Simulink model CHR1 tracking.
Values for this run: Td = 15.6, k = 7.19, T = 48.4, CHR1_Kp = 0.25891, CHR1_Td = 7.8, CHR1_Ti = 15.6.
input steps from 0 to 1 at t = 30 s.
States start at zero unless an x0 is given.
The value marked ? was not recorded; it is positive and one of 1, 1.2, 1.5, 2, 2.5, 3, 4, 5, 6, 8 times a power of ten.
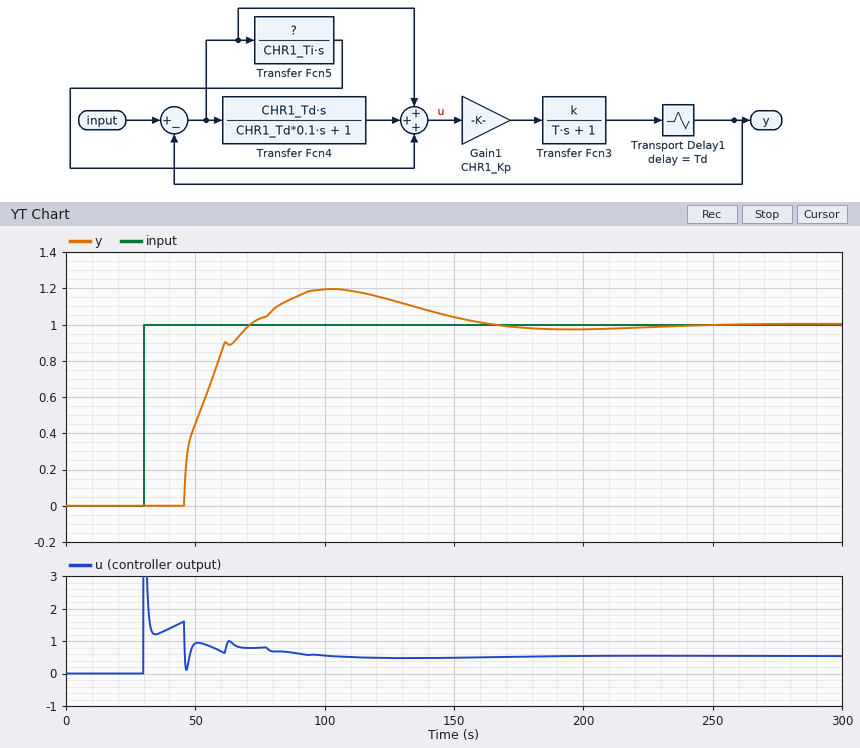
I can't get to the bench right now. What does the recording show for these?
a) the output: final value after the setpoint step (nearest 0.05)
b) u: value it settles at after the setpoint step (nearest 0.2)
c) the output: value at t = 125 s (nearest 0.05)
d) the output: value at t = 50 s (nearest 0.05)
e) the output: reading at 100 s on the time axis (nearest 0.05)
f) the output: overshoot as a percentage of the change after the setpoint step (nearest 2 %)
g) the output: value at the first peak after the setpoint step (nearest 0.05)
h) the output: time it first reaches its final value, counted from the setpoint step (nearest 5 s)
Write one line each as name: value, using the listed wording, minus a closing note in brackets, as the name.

the output: final value after the setpoint step: 1.00
u: value it settles at after the setpoint step: 0.6
the output: value at t = 125 s: 1.15
the output: value at t = 50 s: 0.45
the output: reading at 100 s on the time axis: 1.20
the output: overshoot as a percentage of the change after the setpoint step: 20 %
the output: value at the first peak after the setpoint step: 1.20
the output: time it first reaches its final value, counted from the setpoint step: 40 s
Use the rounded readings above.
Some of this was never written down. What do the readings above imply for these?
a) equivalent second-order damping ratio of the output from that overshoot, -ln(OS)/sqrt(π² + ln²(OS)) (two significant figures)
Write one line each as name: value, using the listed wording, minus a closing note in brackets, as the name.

equivalent second-order damping ratio of the output from that overshoot, -ln(OS)/sqrt(π² + ln²(OS)): 0.46
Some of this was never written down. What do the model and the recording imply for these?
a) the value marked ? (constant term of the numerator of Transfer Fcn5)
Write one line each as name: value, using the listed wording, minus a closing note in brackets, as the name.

the value marked ?: 0.6
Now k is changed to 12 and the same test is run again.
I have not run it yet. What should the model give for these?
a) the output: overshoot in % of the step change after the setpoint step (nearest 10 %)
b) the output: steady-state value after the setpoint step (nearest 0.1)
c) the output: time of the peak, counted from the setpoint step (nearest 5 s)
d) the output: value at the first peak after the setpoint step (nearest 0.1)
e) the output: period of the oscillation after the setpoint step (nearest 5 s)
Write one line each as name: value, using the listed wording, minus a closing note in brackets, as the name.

the output: overshoot in % of the step change after the setpoint step: 50 %
the output: steady-state value after the setpoint step: 1.0
the output: time of the peak, counted from the setpoint step: 30 s
the output: value at the first peak after the setpoint step: 1.5
the output: period of the oscillation after the setpoint step: 35 s
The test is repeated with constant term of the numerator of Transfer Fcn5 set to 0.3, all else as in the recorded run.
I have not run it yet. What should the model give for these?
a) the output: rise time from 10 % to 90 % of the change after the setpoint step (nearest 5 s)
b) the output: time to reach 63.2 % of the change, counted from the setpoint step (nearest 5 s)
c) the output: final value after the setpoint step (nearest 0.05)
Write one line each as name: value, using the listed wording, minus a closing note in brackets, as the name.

the output: rise time from 10 % to 90 % of the change after the setpoint step: 45 s
the output: time to reach 63.2 % of the change, counted from the setpoint step: 25 s
the output: final value after the setpoint step: 1.00
